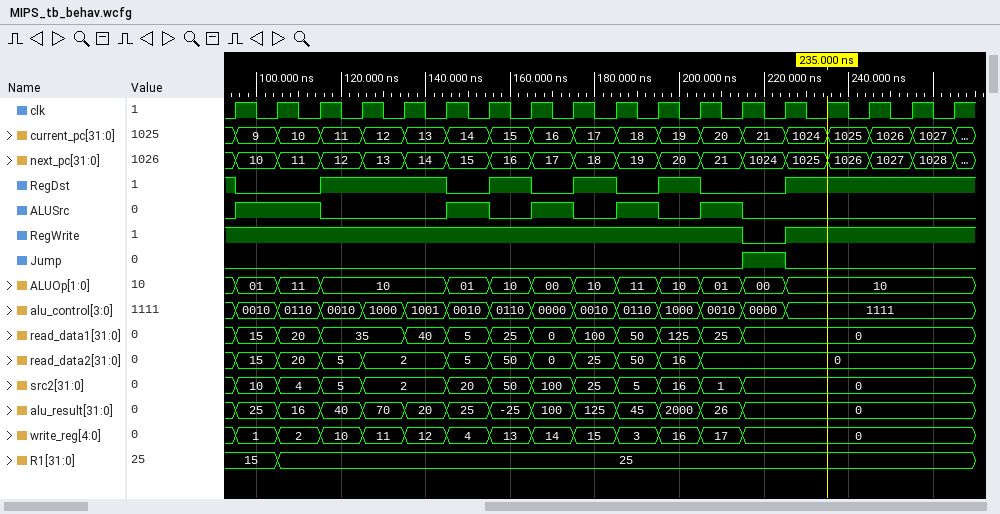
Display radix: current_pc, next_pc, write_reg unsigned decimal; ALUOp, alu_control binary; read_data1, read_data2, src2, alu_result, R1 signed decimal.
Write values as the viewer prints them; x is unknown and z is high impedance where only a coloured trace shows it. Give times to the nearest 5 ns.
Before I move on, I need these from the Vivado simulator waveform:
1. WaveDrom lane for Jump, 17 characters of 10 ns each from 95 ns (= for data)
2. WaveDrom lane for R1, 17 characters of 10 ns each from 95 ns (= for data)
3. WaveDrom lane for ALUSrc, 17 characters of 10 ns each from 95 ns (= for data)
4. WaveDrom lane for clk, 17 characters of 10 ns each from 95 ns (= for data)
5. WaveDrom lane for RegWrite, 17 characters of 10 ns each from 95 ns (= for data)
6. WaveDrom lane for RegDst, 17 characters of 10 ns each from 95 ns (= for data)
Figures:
{name: 'Jump', wave: '0...........10...'}
{name: 'R1', wave: '==...............', data: '15 25'}
{name: 'ALUSrc', wave: '1.0..10101010....'}
{name: 'clk', wave: 'p................'}
{name: 'RegWrite', wave: '1...........01...'}
{name: 'RegDst', wave: '0.1..0101010.1...'}
